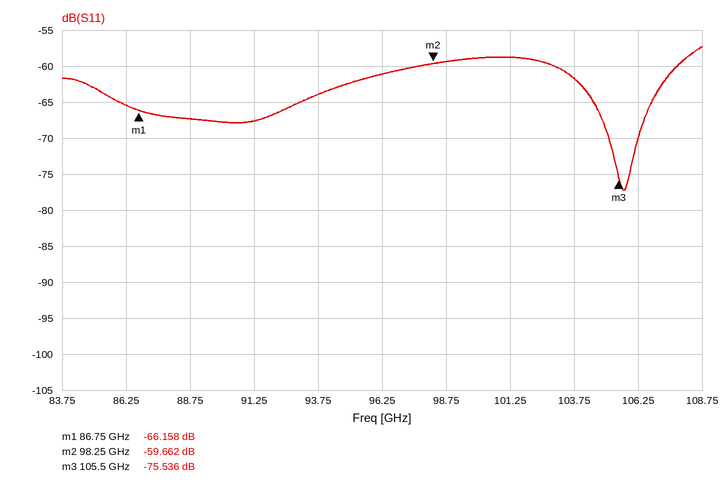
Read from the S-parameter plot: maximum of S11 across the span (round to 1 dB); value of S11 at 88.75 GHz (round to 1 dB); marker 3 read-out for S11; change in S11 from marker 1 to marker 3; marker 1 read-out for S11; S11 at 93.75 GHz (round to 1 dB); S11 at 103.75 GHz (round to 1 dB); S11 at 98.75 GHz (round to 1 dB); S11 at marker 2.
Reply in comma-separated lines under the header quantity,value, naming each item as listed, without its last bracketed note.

quantity,value
maximum of S11 across the span,-57 dB
value of S11 at 88.75 GHz,-67 dB
marker 3 read-out for S11,-75.536 dB
change in S11 from marker 1 to marker 3,-9.378 dB
marker 1 read-out for S11,-66.158 dB
S11 at 93.75 GHz,-64 dB
S11 at 103.75 GHz,-62 dB
S11 at 98.75 GHz,-59 dB
S11 at marker 2,-59.662 dB
